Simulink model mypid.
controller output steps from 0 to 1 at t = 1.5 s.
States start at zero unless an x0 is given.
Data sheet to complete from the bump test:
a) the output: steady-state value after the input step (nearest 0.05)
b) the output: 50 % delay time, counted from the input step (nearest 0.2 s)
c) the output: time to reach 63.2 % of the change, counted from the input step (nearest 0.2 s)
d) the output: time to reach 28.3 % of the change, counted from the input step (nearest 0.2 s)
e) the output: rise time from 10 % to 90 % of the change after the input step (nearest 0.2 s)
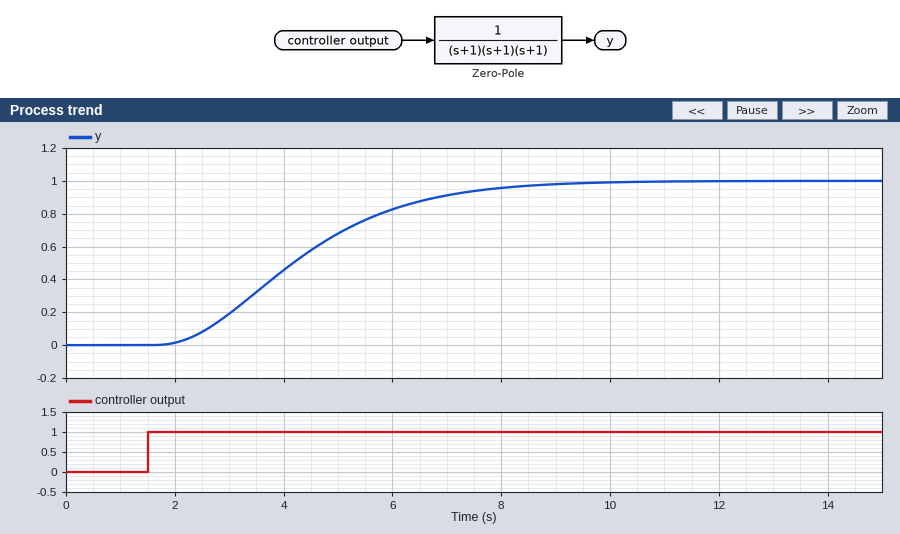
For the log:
1.00
2.6 s
3.2 s
1.8 s
4.2 s
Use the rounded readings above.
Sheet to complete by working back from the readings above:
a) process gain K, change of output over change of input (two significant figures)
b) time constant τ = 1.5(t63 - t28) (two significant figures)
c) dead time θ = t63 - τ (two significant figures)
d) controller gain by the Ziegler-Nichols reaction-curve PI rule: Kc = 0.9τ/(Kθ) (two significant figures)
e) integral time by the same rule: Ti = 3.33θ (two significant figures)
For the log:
1.0
2.1 s
1.1 s
1.7
3.7 s
